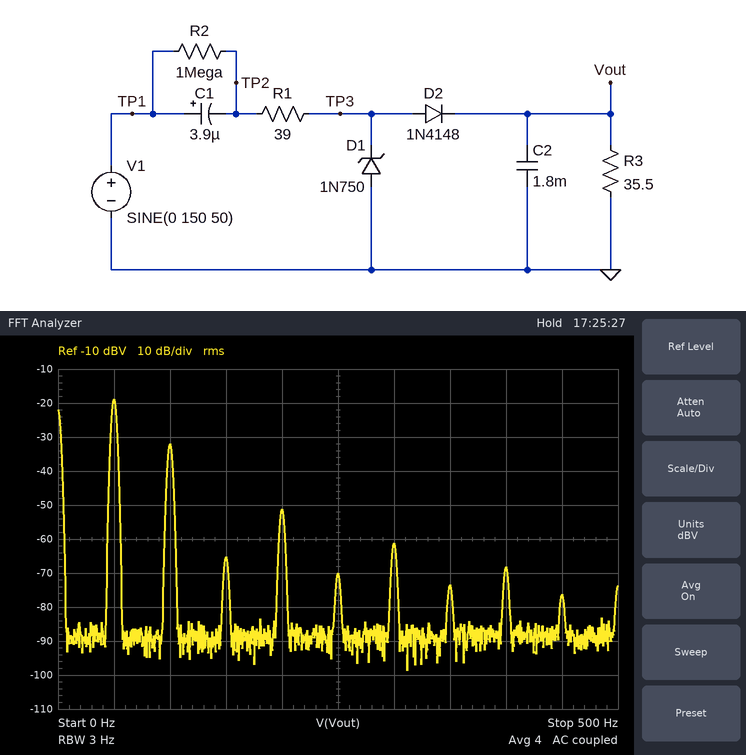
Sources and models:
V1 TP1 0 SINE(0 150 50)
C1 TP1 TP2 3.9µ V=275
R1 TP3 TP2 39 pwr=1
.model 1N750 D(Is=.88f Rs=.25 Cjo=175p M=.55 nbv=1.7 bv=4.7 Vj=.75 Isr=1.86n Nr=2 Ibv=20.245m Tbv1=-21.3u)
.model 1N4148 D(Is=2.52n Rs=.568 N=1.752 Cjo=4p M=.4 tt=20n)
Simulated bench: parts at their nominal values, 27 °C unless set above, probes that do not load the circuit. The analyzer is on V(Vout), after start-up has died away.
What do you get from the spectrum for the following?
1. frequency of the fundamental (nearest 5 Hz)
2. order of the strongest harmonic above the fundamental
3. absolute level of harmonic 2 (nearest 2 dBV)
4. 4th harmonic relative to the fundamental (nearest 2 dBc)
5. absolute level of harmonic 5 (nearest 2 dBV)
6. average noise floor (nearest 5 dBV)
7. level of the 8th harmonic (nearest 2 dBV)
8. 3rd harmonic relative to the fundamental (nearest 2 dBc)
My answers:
50 Hz
2
-32 dBV
-32 dBc
-70 dBV
-90 dBV
-68 dBV
-46 dBc
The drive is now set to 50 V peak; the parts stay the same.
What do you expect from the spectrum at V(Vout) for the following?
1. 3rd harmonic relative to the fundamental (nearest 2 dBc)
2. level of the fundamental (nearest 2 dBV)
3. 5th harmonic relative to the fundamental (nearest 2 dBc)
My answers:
-42 dBc
-28 dBV
-46 dBc
